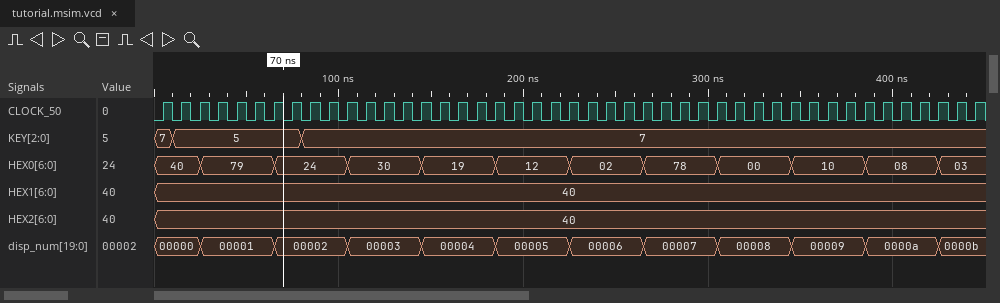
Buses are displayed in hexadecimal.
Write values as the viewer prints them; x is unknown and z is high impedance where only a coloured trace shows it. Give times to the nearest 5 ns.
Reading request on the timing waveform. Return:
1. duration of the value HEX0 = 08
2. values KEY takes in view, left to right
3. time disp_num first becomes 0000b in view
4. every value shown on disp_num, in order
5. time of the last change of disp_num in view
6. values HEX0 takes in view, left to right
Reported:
40 ns
7, 5, 7
425 ns
00000, 00001, 00002, 00003, 00004, 00005, 00006, 00007, 00008, 00009, 0000a, 0000b
425 ns
40, 79, 24, 30, 19, 12, 02, 78, 00, 10, 08, 03
